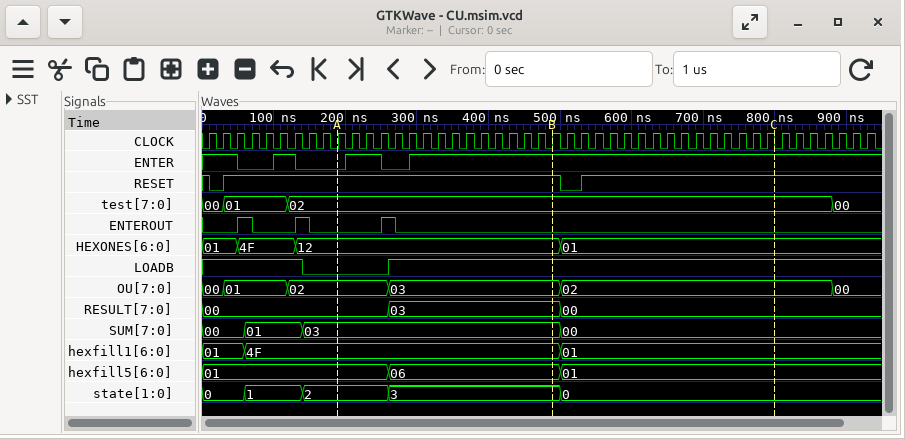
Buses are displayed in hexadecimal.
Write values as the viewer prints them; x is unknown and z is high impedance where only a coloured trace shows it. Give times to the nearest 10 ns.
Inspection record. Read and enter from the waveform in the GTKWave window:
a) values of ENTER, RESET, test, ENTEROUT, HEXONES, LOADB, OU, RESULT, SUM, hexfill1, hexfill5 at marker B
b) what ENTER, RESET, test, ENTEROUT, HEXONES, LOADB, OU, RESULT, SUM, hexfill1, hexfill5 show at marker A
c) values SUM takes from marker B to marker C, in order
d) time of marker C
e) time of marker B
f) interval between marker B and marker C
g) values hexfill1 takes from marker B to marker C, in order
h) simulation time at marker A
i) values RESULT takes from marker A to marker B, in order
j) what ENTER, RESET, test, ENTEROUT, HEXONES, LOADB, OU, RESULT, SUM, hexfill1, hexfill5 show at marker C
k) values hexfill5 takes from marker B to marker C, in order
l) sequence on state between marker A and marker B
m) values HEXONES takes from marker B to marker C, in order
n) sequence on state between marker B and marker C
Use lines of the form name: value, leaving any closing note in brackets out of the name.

values of ENTER, RESET, test, ENTEROUT, HEXONES, LOADB, OU, RESULT, SUM, hexfill1, hexfill5 at marker B: ENTER=1, RESET=1, test=02, ENTEROUT=0, HEXONES=12, LOADB=1, OU=03, RESULT=03, SUM=03, hexfill1=4F, hexfill5=06
what ENTER, RESET, test, ENTEROUT, HEXONES, LOADB, OU, RESULT, SUM, hexfill1, hexfill5 show at marker A: ENTER=0, RESET=1, test=02, ENTEROUT=0, HEXONES=12, LOADB=0, OU=02, RESULT=00, SUM=03, hexfill1=4F, hexfill5=01
values SUM takes from marker B to marker C, in order: 03, 00
time of marker C: 800 ns
time of marker B: 490 ns
interval between marker B and marker C: 310 ns
values hexfill1 takes from marker B to marker C, in order: 4F, 01
simulation time at marker A: 190 ns
values RESULT takes from marker A to marker B, in order: 00, 03
what ENTER, RESET, test, ENTEROUT, HEXONES, LOADB, OU, RESULT, SUM, hexfill1, hexfill5 show at marker C: ENTER=1, RESET=1, test=02, ENTEROUT=0, HEXONES=01, LOADB=1, OU=02, RESULT=00, SUM=00, hexfill1=01, hexfill5=01
values hexfill5 takes from marker B to marker C, in order: 06, 01
sequence on state between marker A and marker B: 2, 3
values HEXONES takes from marker B to marker C, in order: 12, 01
sequence on state between marker B and marker C: 3, 0
